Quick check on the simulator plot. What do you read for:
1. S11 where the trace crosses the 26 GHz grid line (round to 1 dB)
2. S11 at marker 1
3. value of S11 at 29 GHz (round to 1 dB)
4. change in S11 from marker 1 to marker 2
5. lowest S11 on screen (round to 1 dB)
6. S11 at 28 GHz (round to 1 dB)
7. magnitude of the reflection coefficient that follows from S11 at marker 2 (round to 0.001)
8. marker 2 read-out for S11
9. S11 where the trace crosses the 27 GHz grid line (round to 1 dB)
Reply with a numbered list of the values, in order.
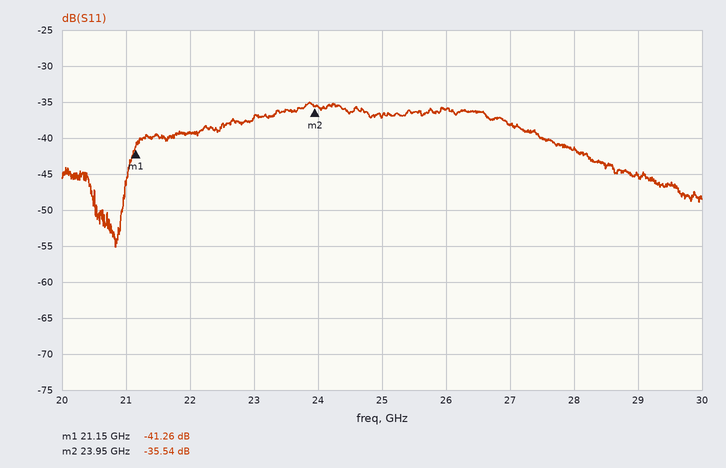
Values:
1. -36 dB
2. -41.26 dB
3. -45 dB
4. 5.72 dB
5. -55 dB
6. -41 dB
7. 0.017
8. -35.54 dB
9. -38 dB
